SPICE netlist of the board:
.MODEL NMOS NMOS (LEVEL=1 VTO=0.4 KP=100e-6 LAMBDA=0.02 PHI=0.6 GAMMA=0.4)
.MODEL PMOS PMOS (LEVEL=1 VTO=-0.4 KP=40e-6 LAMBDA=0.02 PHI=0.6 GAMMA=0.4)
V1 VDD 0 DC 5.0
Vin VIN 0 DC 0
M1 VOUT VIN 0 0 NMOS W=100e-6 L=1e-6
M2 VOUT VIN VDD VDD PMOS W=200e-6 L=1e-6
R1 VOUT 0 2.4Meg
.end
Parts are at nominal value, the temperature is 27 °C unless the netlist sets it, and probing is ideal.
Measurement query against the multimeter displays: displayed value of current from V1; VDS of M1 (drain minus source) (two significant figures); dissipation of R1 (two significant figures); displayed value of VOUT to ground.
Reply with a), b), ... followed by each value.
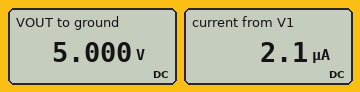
a) 2.1 µA
b) 5.0 V
c) 10 µW
d) 5.000 V
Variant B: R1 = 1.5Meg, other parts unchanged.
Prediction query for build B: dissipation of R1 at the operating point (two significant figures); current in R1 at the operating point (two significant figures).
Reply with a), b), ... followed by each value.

a) 17 µW
b) 3.3 µA
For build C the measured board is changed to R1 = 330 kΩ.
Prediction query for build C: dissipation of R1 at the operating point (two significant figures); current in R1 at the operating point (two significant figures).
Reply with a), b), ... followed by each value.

a) 76 µW
b) 15 µA
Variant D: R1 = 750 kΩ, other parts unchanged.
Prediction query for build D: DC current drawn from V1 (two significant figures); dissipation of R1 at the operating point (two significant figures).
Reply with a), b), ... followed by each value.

a) 6.7 µA
b) 33 µW
